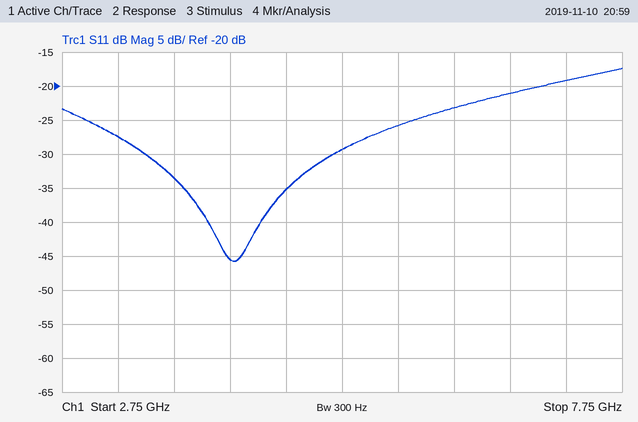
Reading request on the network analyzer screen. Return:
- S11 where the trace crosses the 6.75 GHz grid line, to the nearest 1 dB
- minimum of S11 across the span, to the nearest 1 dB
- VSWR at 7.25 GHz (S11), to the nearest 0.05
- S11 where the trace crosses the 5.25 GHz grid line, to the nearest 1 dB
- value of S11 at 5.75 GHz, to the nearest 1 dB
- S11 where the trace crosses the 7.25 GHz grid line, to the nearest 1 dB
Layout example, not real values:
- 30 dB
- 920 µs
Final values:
- -21 dB
- -46 dB
- 1.25
- -29 dB
- -26 dB
- -19 dB
